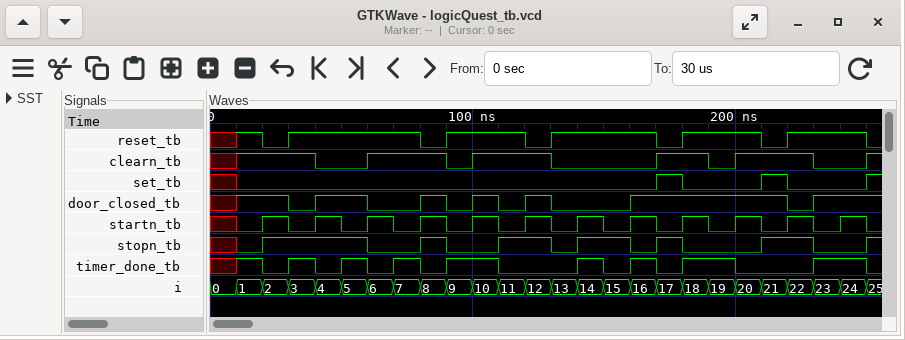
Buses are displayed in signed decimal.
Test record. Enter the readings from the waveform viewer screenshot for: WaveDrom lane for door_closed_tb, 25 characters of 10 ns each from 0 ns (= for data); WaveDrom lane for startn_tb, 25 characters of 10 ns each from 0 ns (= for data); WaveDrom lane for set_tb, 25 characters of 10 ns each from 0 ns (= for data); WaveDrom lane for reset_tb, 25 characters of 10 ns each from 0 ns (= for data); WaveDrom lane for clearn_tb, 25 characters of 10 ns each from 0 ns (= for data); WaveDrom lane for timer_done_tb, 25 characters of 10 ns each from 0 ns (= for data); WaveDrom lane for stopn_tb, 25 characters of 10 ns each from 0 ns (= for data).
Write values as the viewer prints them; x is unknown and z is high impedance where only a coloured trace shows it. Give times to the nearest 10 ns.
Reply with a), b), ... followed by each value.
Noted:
a) {name: 'door_closed_tb', wave: 'x1.01.0.101010..1.....01.'}
b) {name: 'startn_tb', wave: 'x010101010101010101010101'}
c) {name: 'set_tb', wave: 'x0...............10..10..'}
d) {name: 'reset_tb', wave: 'x101....01..01...01..01..'}
e) {name: 'clearn_tb', wave: 'x1..0.1..01..0...1.01..0.'}
f) {name: 'timer_done_tb', wave: 'x101010101.0..10101.0..1.'}
g) {name: 'stopn_tb', wave: 'x01...0.10.1.01.010..1.0.'}
